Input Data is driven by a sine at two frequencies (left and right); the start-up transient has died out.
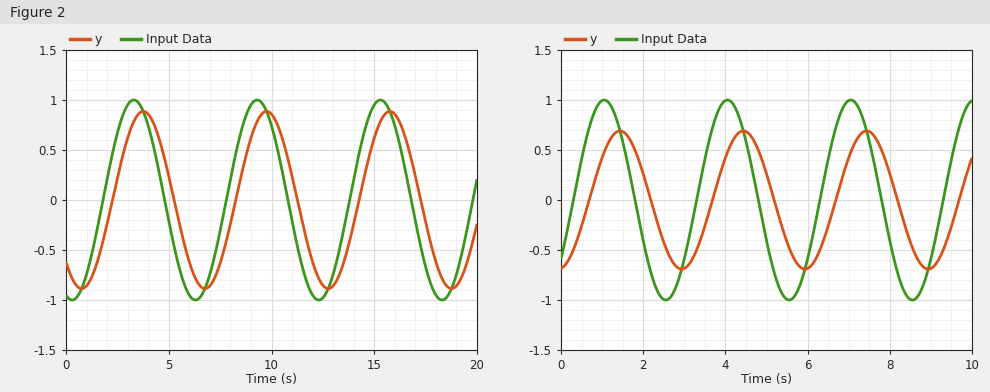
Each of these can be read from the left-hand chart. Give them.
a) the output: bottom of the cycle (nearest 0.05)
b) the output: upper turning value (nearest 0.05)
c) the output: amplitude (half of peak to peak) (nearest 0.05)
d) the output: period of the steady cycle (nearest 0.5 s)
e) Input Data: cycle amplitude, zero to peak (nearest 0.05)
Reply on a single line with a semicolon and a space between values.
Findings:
-0.90; 0.90; 0.90; 6.0 s; 1.00
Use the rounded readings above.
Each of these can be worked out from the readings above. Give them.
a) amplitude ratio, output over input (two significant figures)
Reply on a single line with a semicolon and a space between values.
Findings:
0.90
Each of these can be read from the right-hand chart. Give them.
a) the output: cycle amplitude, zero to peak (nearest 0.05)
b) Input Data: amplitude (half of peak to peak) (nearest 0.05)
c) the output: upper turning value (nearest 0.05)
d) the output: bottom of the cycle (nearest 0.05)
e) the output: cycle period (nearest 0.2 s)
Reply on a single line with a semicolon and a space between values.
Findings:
0.70; 1.00; 0.70; -0.70; 3.0 s
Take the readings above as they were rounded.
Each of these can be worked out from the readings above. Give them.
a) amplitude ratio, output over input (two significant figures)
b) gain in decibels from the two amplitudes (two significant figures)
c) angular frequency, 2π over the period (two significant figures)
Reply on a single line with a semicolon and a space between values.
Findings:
0.70; -3.1 dB; 2.1 rad/s
